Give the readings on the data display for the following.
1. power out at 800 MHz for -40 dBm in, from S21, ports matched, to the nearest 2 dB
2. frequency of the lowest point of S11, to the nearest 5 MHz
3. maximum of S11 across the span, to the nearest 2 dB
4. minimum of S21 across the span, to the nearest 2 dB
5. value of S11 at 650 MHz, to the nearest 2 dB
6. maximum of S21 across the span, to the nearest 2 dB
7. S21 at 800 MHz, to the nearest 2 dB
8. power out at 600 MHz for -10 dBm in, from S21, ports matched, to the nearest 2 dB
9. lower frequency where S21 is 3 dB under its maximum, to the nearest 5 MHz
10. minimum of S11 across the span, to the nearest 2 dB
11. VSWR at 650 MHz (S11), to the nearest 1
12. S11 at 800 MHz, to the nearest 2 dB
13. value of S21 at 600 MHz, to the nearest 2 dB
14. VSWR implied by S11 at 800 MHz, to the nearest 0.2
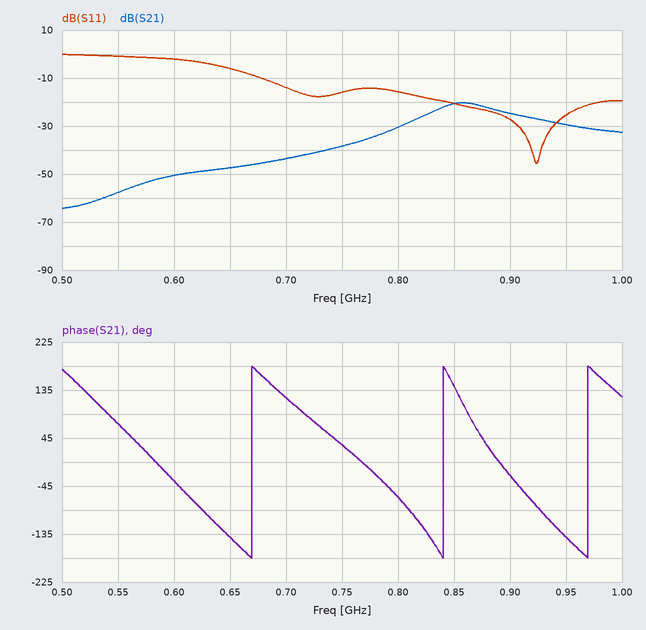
-70 dBm
925 MHz
0 dB
-64 dB
-6 dB
-20 dB
-30 dB
-60 dBm
835 MHz
-46 dB
3
-16 dB
-50 dB
1.4
